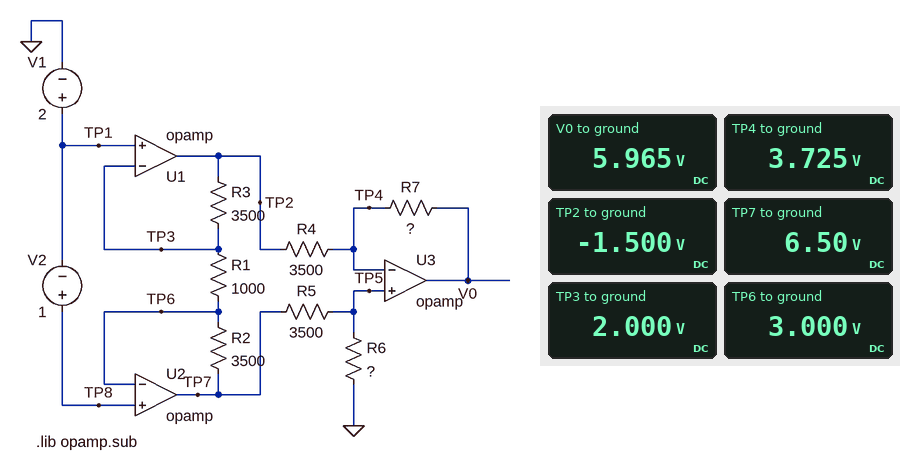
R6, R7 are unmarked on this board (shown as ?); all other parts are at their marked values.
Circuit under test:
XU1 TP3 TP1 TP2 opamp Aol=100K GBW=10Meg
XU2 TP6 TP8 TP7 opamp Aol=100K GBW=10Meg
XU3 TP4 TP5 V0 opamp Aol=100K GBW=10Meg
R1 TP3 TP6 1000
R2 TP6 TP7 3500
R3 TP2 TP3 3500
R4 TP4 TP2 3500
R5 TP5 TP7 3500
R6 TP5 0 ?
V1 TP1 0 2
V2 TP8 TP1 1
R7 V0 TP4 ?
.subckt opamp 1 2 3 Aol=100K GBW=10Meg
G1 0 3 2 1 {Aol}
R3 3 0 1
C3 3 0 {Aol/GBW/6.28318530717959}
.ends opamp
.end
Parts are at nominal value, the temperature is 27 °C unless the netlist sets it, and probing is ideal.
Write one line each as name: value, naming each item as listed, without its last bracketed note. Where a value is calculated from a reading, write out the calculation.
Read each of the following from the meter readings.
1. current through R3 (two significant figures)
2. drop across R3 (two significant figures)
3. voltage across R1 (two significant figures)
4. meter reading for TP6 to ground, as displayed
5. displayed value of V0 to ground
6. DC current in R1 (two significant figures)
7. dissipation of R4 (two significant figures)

current through R3: (2 V - (-1.5 V)) / 3.5 kΩ = 1.0 mA
drop across R3: 2 V - (-1.5 V) = 3.5 V
voltage across R1: 3 V - 2 V = 1.0 V
meter reading for TP6 to ground, as displayed: 3.000 V
displayed value of V0 to ground: 5.965 V
DC current in R1: (3 V - 2 V) / 1 kΩ = 1.0 mA
dissipation of R4: (3.725 V - (-1.5 V))^2 / 3.5 kΩ = 7.8 mW
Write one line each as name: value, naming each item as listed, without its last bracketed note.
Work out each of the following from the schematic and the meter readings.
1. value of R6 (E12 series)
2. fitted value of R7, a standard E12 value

value of R6: 4.7 kΩ
fitted value of R7, a standard E12 value: 1.5 kΩ
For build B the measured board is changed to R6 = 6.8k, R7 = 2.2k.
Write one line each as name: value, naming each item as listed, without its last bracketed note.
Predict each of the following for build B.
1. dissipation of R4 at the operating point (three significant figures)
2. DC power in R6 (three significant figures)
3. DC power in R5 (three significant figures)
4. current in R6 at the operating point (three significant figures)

dissipation of R4 at the operating point: 9.58 mW
DC power in R6: 2.71 mW
DC power in R5: 1.39 mW
current in R6 at the operating point: 631 µA
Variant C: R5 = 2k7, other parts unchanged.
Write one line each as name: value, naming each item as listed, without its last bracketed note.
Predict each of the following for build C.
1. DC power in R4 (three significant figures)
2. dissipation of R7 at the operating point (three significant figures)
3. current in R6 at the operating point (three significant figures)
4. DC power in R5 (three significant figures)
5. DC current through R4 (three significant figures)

DC power in R4: 9.05 mW
dissipation of R7 at the operating point: 3.88 mW
current in R6 at the operating point: 878 µA
DC power in R5: 2.08 mW
DC current through R4: 1.61 mA
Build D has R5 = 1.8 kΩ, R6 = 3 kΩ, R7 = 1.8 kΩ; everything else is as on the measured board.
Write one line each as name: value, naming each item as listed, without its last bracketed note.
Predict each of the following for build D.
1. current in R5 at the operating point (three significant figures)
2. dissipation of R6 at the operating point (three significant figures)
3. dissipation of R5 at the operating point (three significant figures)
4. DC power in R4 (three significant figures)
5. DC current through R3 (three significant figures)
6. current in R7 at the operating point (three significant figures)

current in R5 at the operating point: 1.35 mA
dissipation of R6 at the operating point: 5.50 mW
dissipation of R5 at the operating point: 3.30 mW
DC power in R4: 8.84 mW
DC current through R3: 1.00 mA
current in R7 at the operating point: 1.59 mA
